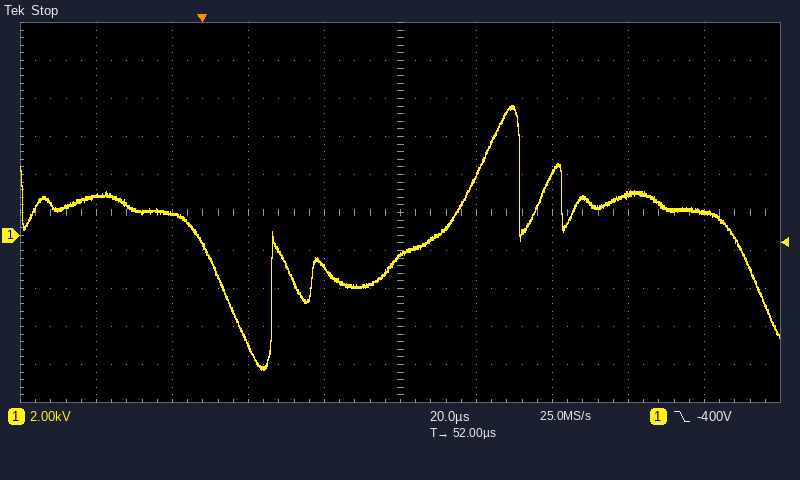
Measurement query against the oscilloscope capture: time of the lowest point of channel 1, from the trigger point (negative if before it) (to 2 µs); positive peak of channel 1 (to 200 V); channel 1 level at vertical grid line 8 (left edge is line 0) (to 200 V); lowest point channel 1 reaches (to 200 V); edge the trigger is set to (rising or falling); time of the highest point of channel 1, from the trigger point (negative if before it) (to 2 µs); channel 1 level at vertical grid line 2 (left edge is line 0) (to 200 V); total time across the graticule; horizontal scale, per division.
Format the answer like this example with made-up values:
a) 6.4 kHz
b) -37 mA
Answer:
a) +16 µs
b) 6.8 kV
c) 2.2 kV
d) -7.0 kV
e) falling
f) +82 µs
g) 1.2 kV
h) 200 µs
i) 20 µs
